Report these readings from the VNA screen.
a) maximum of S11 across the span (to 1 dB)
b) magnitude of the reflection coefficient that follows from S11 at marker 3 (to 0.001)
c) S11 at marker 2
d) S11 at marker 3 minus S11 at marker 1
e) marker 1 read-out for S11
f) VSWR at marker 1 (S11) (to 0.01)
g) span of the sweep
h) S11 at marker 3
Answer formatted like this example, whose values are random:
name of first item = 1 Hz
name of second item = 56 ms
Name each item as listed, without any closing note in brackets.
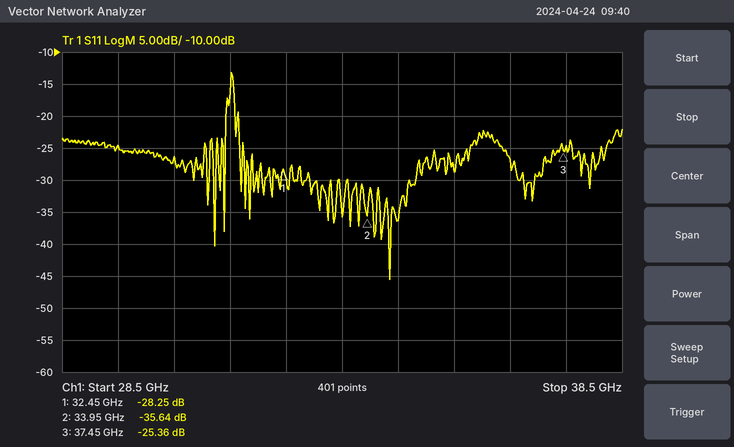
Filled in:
maximum of S11 across the span = -13 dB
magnitude of the reflection coefficient that follows from S11 at marker 3 = 0.054
S11 at marker 2 = -35.64 dB
S11 at marker 3 minus S11 at marker 1 = 2.89 dB
marker 1 read-out for S11 = -28.25 dB
VSWR at marker 1 (S11) = 1.08
span of the sweep = 10 GHz
S11 at marker 3 = -25.36 dB
